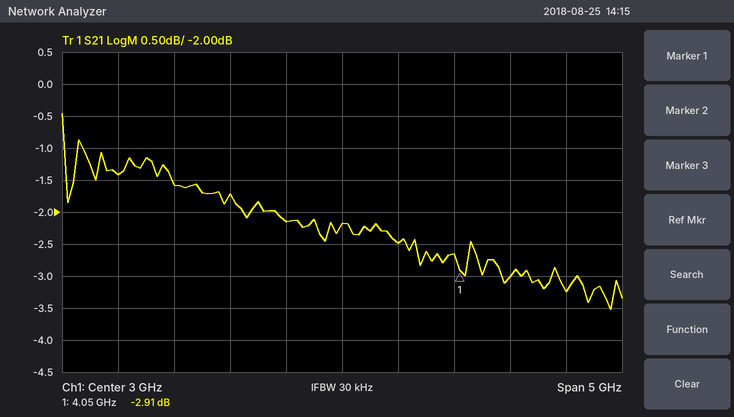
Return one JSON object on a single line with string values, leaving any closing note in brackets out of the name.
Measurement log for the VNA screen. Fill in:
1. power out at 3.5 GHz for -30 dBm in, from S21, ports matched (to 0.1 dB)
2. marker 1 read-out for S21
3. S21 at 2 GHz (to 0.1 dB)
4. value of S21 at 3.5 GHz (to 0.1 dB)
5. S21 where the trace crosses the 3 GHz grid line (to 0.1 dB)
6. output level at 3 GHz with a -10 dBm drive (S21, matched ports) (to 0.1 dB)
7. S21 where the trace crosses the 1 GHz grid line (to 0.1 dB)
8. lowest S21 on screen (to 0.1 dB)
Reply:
{"power out at 3.5 GHz for -30 dBm in, from S21, ports matched": "-32.5 dBm", "marker 1 read-out for S21": "-2.91 dB", "S21 at 2 GHz": "-1.7 dB", "value of S21 at 3.5 GHz": "-2.5 dB", "S21 where the trace crosses the 3 GHz grid line": "-2.2 dB", "output level at 3 GHz with a -10 dBm drive (S21, matched ports)": "-12.2 dBm", "S21 where the trace crosses the 1 GHz grid line": "-1.4 dB", "lowest S21 on screen": "-3.5 dB"}
